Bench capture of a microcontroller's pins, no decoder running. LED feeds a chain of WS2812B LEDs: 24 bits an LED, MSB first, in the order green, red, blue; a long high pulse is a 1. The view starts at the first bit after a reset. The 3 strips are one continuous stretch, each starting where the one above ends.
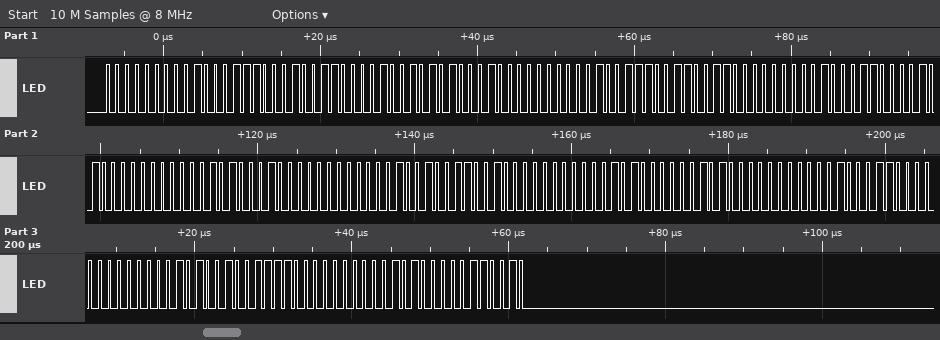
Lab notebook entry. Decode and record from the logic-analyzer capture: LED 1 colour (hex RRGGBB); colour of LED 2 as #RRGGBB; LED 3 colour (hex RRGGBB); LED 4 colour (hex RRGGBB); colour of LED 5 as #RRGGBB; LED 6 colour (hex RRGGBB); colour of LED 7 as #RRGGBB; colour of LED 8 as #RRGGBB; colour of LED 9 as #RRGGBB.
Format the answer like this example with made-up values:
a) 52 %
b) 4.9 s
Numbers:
a) #470013
b) #510900
c) #332700
d) #144600
e) #005109
f) #003228
g) #001446
h) #0A004F
i) #280032
